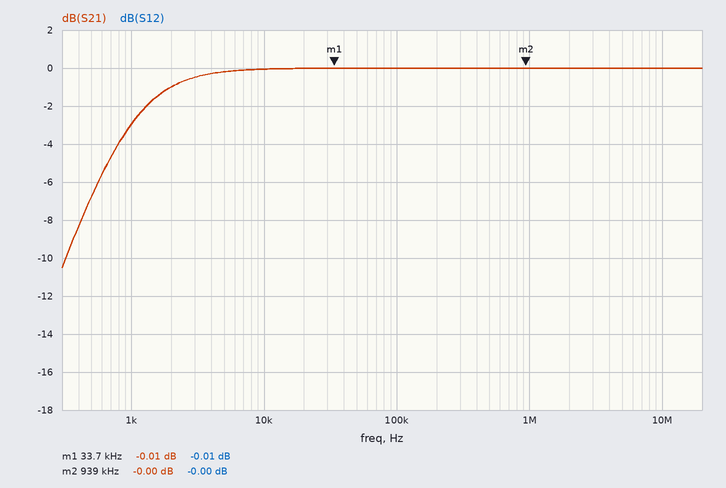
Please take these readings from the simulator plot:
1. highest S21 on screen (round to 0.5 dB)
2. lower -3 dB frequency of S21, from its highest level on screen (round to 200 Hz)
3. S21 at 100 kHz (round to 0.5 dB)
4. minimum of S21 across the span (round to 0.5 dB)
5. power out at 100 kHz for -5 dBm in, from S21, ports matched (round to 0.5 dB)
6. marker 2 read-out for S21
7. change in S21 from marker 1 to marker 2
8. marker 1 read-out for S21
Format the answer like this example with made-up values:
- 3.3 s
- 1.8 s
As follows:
- 0.0 dB
- 1.0 kHz
- 0.0 dB
- -10.5 dB
- -5.0 dBm
- -0.00 dB
- 0.01 dB
- -0.01 dB
